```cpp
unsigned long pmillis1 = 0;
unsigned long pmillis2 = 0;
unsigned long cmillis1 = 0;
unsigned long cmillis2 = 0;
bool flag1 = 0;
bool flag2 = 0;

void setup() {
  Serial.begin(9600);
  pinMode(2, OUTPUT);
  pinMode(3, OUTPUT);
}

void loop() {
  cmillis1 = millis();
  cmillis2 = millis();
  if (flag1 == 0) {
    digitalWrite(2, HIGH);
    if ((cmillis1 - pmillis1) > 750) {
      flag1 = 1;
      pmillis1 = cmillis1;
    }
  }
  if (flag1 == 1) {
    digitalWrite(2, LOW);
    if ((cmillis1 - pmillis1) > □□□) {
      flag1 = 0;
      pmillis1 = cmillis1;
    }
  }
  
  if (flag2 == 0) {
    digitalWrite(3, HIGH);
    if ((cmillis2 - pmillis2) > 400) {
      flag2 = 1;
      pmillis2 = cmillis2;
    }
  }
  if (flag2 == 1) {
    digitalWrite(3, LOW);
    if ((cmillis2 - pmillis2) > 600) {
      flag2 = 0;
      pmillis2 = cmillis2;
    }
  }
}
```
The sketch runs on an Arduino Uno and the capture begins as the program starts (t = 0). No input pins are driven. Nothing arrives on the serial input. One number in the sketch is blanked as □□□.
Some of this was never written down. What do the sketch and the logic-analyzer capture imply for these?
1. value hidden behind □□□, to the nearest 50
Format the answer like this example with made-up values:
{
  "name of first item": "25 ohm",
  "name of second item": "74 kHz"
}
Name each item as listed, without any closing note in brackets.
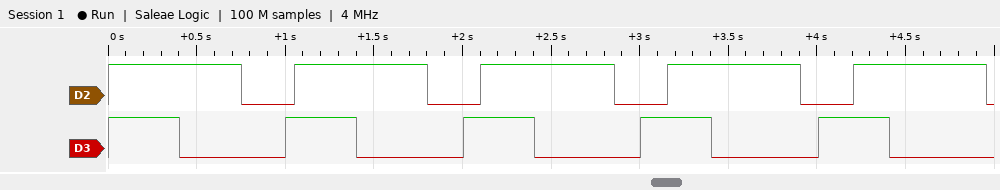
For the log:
{
  "value hidden behind □□□, to the nearest 50": "300"
}
